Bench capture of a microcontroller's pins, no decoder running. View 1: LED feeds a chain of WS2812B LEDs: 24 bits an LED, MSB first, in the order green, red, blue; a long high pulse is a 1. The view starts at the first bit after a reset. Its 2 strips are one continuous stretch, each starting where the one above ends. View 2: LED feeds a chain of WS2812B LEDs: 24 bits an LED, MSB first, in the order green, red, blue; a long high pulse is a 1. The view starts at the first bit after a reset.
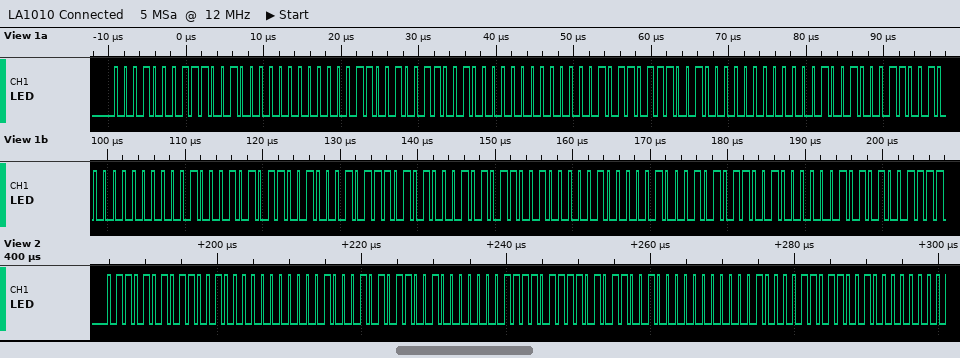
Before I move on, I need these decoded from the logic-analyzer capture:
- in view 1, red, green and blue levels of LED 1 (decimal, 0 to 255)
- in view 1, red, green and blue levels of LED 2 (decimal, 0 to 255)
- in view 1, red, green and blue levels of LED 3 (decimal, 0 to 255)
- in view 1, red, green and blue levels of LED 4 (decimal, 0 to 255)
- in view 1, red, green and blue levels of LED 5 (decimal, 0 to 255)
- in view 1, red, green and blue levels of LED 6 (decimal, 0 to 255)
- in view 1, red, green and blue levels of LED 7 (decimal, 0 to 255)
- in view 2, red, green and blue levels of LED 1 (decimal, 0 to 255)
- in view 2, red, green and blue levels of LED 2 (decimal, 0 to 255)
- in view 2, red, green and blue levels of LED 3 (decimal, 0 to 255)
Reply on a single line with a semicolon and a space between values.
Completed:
200, 17, 0; 200, 100, 0; 200, 45, 0; 200, 72, 0; 200, 138, 186; 200, 138, 32; 200, 138, 21; 200, 106, 0; 200, 138, 15; 200, 122, 0
